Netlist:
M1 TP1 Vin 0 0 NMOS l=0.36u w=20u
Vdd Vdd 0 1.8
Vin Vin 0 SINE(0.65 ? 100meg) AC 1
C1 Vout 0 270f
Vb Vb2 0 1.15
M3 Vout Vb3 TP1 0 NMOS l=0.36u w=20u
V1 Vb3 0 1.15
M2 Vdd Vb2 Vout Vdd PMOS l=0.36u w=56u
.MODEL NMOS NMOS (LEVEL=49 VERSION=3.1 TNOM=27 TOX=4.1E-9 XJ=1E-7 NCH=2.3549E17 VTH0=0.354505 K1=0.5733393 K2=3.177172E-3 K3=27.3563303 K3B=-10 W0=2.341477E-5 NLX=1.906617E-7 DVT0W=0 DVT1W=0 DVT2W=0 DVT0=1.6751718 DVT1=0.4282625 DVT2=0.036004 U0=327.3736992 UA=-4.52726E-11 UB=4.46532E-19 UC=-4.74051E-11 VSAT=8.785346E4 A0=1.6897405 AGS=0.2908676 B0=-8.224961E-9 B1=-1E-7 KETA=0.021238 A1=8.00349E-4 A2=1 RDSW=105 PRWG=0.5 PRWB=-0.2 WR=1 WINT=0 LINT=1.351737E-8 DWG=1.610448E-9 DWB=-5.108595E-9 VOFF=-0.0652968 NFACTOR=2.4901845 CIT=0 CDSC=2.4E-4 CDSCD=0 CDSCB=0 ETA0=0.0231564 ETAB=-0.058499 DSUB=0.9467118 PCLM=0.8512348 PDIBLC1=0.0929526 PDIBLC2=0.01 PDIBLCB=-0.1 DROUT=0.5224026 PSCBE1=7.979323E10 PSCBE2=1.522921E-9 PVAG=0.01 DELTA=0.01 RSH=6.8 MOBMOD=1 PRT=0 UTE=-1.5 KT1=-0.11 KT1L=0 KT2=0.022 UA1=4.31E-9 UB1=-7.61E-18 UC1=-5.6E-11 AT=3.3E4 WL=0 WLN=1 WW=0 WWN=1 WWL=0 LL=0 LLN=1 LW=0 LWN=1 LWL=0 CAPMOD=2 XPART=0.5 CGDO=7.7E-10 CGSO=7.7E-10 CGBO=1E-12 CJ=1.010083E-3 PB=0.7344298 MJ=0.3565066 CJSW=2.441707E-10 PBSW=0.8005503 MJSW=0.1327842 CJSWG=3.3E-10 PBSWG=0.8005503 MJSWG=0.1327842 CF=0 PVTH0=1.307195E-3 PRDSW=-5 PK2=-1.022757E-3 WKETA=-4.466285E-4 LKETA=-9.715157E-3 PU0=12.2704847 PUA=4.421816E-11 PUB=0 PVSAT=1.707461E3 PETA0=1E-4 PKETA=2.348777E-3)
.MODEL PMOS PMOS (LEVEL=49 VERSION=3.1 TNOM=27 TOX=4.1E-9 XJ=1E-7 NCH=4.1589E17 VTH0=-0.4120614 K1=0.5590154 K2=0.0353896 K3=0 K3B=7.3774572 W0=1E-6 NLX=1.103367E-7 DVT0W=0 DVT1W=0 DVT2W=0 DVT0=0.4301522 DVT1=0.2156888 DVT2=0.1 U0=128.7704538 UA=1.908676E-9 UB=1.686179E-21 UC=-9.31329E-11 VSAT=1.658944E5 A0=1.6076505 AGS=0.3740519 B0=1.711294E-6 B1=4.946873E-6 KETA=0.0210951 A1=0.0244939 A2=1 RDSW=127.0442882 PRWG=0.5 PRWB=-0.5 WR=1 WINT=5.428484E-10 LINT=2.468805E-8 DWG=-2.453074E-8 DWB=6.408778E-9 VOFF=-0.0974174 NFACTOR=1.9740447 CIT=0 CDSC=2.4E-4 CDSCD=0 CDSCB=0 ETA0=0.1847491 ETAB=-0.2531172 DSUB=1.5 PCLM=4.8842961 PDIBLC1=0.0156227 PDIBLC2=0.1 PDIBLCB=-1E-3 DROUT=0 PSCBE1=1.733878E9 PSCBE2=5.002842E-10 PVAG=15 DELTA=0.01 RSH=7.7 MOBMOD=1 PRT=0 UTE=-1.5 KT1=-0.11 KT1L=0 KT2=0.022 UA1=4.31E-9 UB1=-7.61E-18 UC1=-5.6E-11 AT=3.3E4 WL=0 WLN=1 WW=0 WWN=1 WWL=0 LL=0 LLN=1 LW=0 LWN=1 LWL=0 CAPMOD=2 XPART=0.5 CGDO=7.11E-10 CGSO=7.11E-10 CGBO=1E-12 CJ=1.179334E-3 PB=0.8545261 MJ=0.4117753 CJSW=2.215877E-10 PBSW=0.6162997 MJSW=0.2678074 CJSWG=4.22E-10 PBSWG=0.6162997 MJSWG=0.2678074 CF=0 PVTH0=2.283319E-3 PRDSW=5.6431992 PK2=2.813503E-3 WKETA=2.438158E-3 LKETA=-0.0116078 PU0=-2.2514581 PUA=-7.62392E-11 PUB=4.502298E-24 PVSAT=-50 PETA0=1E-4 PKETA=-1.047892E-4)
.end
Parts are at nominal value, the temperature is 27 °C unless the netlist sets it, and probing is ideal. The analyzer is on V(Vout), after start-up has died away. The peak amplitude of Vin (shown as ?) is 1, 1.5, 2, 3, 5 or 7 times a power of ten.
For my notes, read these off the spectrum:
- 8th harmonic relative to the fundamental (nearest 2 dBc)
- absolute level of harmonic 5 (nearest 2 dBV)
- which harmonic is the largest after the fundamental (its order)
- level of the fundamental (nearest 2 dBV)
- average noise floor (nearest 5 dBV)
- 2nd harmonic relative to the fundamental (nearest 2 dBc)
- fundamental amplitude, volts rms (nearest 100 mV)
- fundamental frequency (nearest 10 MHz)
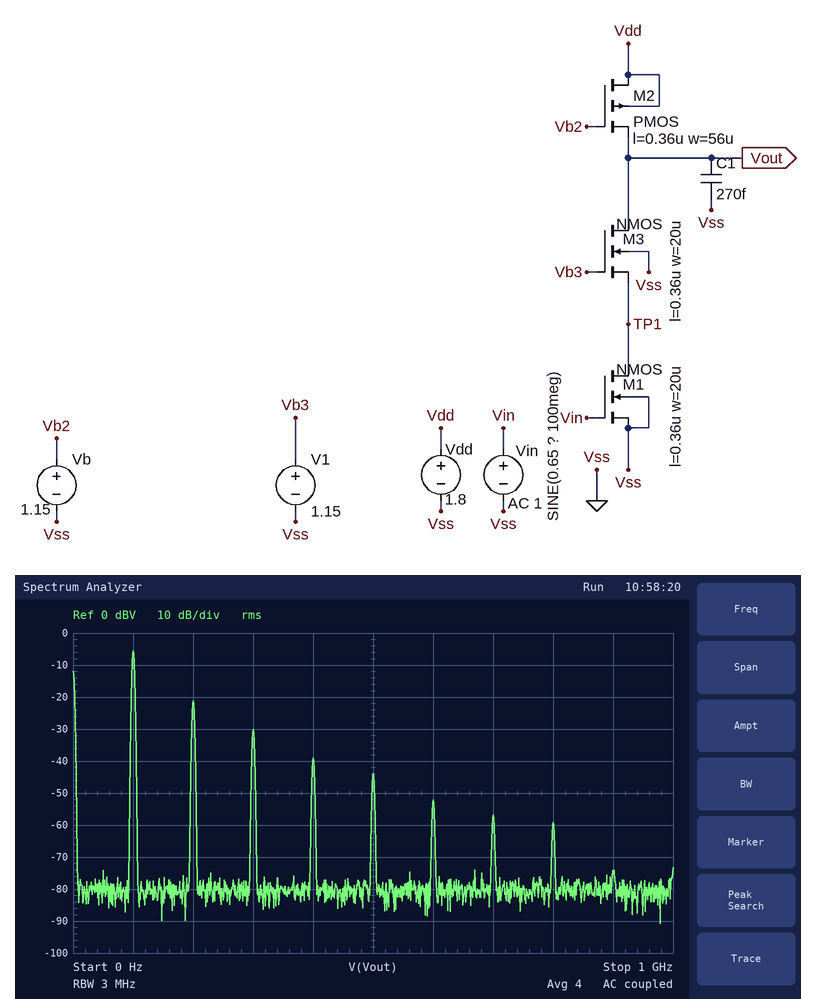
-54 dBc
-44 dBV
2
-6 dBV
-80 dBV
-16 dBc
500 mV
100 MHz
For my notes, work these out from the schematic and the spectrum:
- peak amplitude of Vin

100 mV
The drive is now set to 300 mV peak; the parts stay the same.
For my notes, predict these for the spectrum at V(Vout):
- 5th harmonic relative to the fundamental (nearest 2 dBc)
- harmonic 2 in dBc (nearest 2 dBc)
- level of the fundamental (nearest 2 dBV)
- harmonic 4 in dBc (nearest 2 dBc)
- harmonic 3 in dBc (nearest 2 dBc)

-26 dBc
-12 dBc
-4 dBV
-24 dBc
-18 dBc
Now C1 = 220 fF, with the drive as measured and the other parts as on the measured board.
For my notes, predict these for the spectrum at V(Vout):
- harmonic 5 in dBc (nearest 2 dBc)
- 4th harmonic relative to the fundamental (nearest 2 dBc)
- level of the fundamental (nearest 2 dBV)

-36 dBc
-30 dBc
-4 dBV
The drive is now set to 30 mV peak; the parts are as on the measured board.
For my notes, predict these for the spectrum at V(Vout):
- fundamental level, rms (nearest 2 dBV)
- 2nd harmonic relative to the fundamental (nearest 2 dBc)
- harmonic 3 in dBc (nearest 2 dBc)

-14 dBV
-32 dBc
-60 dBc
